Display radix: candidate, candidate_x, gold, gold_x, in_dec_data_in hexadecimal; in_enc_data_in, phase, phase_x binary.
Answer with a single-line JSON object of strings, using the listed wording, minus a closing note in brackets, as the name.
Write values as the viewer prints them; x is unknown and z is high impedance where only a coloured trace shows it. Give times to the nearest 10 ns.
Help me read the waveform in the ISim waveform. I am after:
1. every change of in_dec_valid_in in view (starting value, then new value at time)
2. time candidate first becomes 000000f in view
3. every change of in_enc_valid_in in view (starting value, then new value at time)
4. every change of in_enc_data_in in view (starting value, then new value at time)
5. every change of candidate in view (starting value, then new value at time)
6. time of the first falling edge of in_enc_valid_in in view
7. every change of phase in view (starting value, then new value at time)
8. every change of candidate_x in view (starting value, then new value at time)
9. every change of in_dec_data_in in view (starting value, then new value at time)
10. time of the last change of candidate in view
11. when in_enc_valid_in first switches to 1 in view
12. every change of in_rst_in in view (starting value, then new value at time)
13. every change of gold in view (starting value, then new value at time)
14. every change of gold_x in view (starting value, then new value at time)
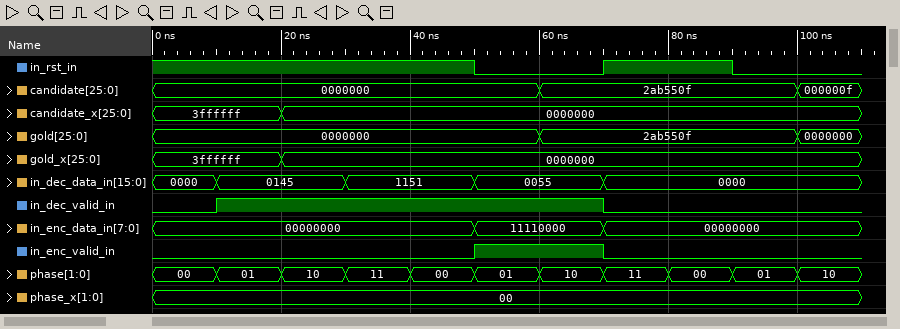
{"every change of in_dec_valid_in in view": "0, 1 at 10 ns, 0 at 70 ns", "time candidate first becomes 000000f in view": "100 ns", "every change of in_enc_valid_in in view": "0, 1 at 50 ns, 0 at 70 ns", "every change of in_enc_data_in in view": "00000000, 11110000 at 50 ns, 00000000 at 70 ns", "every change of candidate in view": "0000000, 2ab550f at 60 ns, 000000f at 100 ns", "time of the first falling edge of in_enc_valid_in in view": "70 ns", "every change of phase in view": "00, 01 at 10 ns, 10 at 20 ns, 11 at 30 ns, 00 at 40 ns, 01 at 50 ns, 10 at 60 ns, 11 at 70 ns, 00 at 80 ns, 01 at 90 ns, 10 at 100 ns", "every change of candidate_x in view": "3ffffff, 0000000 at 20 ns", "every change of in_dec_data_in in view": "0000, 0145 at 10 ns, 1151 at 30 ns, 0055 at 50 ns, 0000 at 70 ns", "time of the last change of candidate in view": "100 ns", "when in_enc_valid_in first switches to 1 in view": "50 ns", "every change of in_rst_in in view": "1, 0 at 50 ns, 1 at 70 ns, 0 at 90 ns", "every change of gold in view": "0000000, 2ab550f at 60 ns, 0000000 at 100 ns", "every change of gold_x in view": "3ffffff, 0000000 at 20 ns"}
